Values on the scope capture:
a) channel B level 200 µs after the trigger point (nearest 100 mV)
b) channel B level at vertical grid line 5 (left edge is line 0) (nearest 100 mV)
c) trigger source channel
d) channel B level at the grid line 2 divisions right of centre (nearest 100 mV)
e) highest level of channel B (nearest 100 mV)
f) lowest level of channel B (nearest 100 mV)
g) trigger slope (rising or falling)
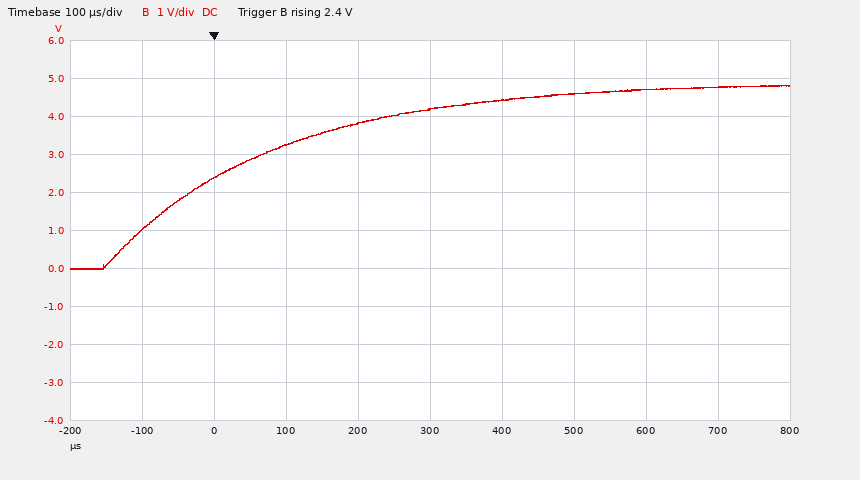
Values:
3.8 V
4.2 V
channel B
4.6 V
4.8 V
0.0 V
rising
